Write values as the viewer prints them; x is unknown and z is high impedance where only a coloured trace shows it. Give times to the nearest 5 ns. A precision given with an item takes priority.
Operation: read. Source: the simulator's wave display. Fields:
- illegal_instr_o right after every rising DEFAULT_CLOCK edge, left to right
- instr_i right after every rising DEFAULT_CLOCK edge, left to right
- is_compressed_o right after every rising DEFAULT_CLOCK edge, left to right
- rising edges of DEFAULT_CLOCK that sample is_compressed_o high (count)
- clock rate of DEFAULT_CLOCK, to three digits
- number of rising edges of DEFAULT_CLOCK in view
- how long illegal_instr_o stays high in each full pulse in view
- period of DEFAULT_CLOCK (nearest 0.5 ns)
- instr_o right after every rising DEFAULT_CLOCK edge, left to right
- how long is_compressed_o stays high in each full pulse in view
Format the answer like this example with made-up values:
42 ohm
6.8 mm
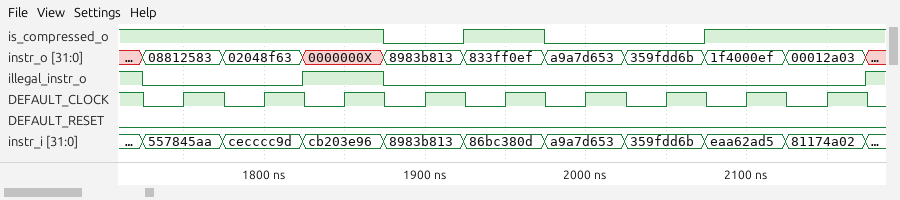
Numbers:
0 0 1 0 0 0 0 0 0
557845aa, cecccc9d, cb203e96, 8983b813, 86bc380d, a9a7d653, 359fdd6b, eaa62ad5, 81174a02
1 1 1 0 1 0 0 1 1
6
20.0 MHz
9
50 ns
50 ns
08812583, 02048f63, 0000000X, 8983b813, 833ff0ef, a9a7d653, 359fdd6b, 1f4000ef, 00012a03
50 ns
